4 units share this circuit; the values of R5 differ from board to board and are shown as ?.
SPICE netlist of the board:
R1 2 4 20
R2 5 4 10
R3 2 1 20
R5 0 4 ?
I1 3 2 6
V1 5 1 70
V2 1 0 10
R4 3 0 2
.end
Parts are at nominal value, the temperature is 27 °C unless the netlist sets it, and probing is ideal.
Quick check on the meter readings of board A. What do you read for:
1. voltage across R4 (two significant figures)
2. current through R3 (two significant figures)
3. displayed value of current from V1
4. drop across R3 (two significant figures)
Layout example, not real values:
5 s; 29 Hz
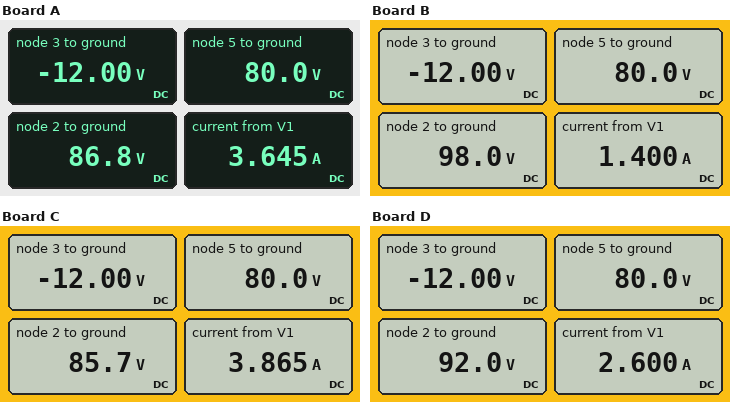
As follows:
12 V; 3.8 A; 3.645 A; 77 V
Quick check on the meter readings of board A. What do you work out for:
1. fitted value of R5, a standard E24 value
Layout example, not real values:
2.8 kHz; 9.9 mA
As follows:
7.5 Ω
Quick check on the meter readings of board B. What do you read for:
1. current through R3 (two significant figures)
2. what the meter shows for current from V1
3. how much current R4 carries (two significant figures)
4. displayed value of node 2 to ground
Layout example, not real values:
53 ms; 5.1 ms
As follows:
4.4 A; 1.400 A; 6.0 A; 98.0 V
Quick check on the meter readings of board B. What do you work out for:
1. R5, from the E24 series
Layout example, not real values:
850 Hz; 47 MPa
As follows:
22 Ω
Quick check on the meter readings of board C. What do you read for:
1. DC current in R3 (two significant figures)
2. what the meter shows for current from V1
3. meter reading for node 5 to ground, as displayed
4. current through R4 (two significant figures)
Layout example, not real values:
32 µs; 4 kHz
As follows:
3.8 A; 3.865 A; 80.0 V; 6.0 A
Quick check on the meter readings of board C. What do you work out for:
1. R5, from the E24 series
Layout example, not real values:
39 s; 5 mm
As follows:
6.8 Ω
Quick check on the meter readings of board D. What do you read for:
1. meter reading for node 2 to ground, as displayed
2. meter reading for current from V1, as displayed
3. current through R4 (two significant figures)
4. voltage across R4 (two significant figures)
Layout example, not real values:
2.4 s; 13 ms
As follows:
92.0 V; 2.600 A; 6.0 A; 12 V
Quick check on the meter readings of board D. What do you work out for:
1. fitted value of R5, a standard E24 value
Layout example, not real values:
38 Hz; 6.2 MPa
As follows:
12 Ω
